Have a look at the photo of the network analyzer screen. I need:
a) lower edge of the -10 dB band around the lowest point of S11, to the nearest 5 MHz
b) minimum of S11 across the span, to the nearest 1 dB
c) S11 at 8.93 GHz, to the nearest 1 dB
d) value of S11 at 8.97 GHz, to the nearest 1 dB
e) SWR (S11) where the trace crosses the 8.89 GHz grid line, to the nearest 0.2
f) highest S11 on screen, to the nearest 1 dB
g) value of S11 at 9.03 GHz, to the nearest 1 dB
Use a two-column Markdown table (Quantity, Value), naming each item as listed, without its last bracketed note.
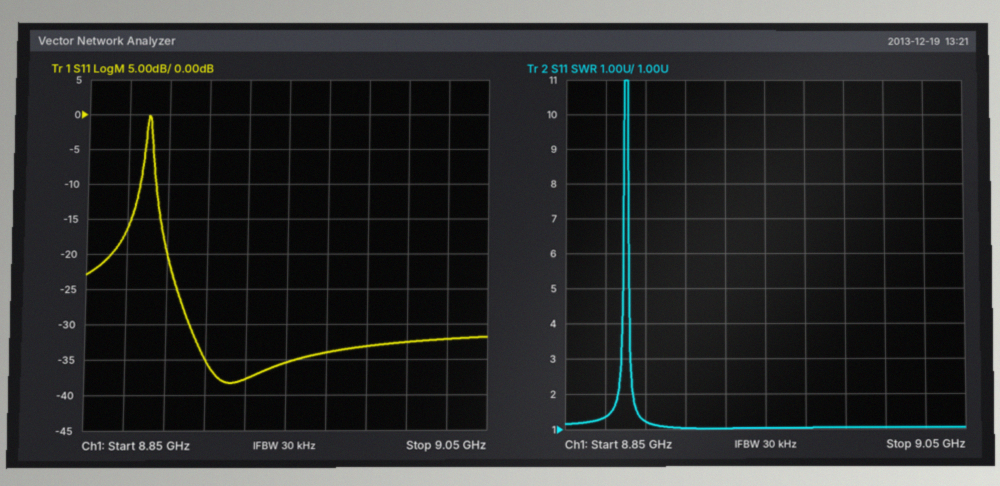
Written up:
| Quantity | Value |
|---|---|
| lower edge of the -10 dB band around the lowest point of S11, to the nearest 5 MHz | 8.885 GHz |
| minimum of S11 across the span, to the nearest 1 dB | -38 dB |
| S11 at 8.93 GHz, to the nearest 1 dB | -38 dB |
| value of S11 at 8.97 GHz, to the nearest 1 dB | -34 dB |
| SWR (S11) where the trace crosses the 8.89 GHz grid line, to the nearest 0.2 | 1.2 |
| highest S11 on screen, to the nearest 1 dB | 0 dB |
| value of S11 at 9.03 GHz, to the nearest 1 dB | -32 dB |
